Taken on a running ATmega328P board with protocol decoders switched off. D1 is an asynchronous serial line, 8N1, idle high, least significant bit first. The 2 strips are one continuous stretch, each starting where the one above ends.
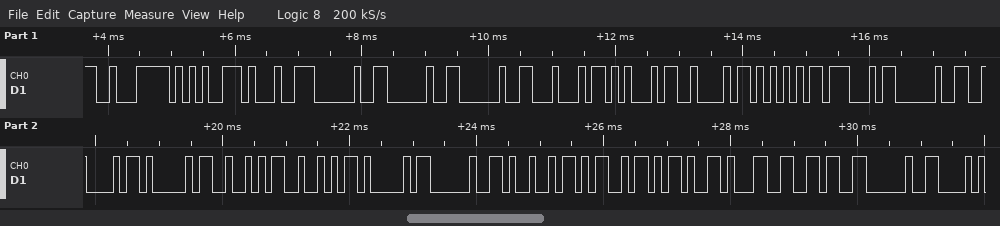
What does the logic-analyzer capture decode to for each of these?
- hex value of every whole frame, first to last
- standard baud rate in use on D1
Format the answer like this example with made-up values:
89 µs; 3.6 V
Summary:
0xE2 0x95 0x91 0x20 0x20 0x20 0x44 0x45 0x42 0x55 0x47 0x20 0x42 0x41 0x52 0x52 0x41 0x20 0x49 0x4D 0x2D 0x31 0x36 0x20; 9600 baud
